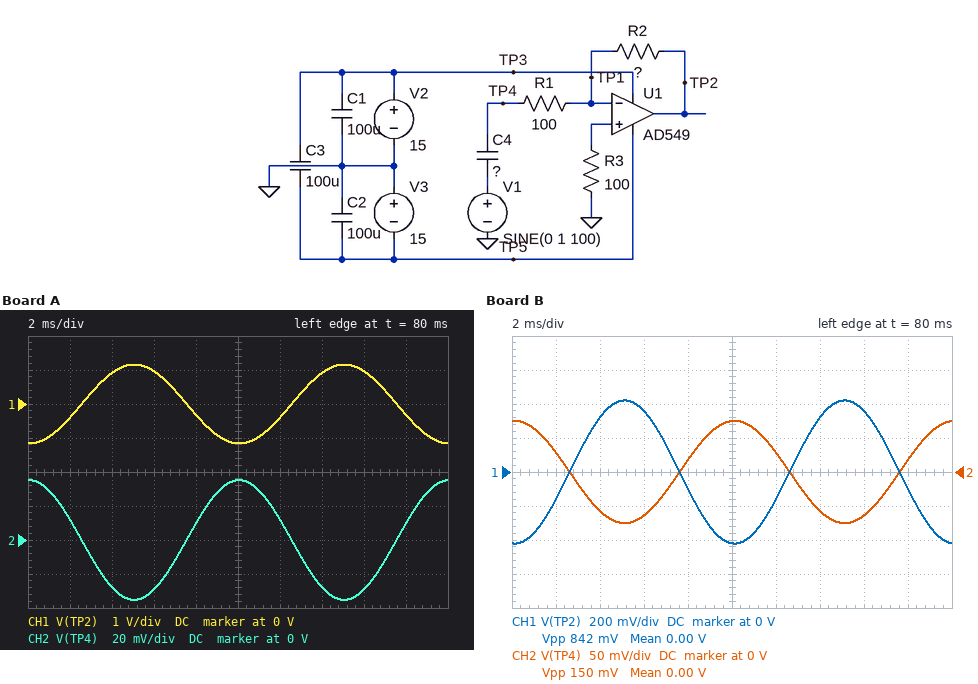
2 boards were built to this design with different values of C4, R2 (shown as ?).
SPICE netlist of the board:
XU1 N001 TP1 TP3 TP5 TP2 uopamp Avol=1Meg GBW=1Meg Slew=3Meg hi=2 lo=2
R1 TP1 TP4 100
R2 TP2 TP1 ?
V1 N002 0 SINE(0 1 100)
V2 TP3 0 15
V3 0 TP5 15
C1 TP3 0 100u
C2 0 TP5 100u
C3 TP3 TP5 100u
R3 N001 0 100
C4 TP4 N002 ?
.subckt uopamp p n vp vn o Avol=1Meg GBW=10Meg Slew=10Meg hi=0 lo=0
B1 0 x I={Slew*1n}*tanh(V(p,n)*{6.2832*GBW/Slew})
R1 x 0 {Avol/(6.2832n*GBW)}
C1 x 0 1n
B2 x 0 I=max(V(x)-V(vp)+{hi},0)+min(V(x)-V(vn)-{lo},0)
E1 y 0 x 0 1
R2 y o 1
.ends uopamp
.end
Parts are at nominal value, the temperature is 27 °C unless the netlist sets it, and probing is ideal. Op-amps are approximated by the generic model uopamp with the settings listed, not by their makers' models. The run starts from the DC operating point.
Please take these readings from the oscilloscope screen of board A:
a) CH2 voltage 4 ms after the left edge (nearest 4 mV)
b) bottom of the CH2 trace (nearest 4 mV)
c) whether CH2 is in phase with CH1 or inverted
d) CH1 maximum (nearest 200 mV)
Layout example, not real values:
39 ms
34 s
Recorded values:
-28 mV
-36 mV
inverted
1.2 V
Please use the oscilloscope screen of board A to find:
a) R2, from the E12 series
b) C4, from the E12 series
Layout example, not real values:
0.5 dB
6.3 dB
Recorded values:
3.3 kΩ
560 nF
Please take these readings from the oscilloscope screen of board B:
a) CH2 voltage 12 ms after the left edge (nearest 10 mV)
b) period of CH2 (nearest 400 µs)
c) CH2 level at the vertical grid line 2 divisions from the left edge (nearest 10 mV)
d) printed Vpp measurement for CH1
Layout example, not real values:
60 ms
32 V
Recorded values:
30 mV
10.0 ms
-60 mV
842 mV
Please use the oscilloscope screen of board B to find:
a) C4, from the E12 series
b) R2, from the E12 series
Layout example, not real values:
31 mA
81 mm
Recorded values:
1.2 µF
560 Ω
